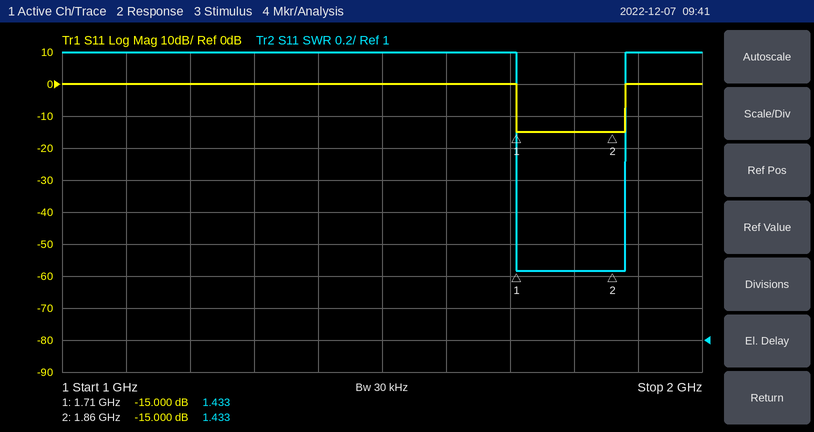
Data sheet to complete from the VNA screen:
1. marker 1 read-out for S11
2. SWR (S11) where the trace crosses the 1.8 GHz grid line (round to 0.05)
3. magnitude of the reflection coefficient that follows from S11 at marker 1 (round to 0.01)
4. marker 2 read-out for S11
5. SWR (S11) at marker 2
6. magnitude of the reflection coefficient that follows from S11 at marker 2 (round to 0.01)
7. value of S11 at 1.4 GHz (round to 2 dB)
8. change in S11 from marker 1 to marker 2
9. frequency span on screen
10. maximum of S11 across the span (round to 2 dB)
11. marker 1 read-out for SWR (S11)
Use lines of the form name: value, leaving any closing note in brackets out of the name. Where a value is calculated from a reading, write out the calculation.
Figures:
marker 1 read-out for S11: -15.000 dB
SWR (S11) where the trace crosses the 1.8 GHz grid line: 1.45
magnitude of the reflection coefficient that follows from S11 at marker 1: 10^(-15/20) ≈ 0.18
marker 2 read-out for S11: -15.000 dB
SWR (S11) at marker 2: 1.433
magnitude of the reflection coefficient that follows from S11 at marker 2: 10^(-15/20) ≈ 0.18
value of S11 at 1.4 GHz: 0 dB
change in S11 from marker 1 to marker 2: -15 − (-15) = 0.000 dB
frequency span on screen: 1 GHz
maximum of S11 across the span: 0 dB
marker 1 read-out for SWR: 1.433
